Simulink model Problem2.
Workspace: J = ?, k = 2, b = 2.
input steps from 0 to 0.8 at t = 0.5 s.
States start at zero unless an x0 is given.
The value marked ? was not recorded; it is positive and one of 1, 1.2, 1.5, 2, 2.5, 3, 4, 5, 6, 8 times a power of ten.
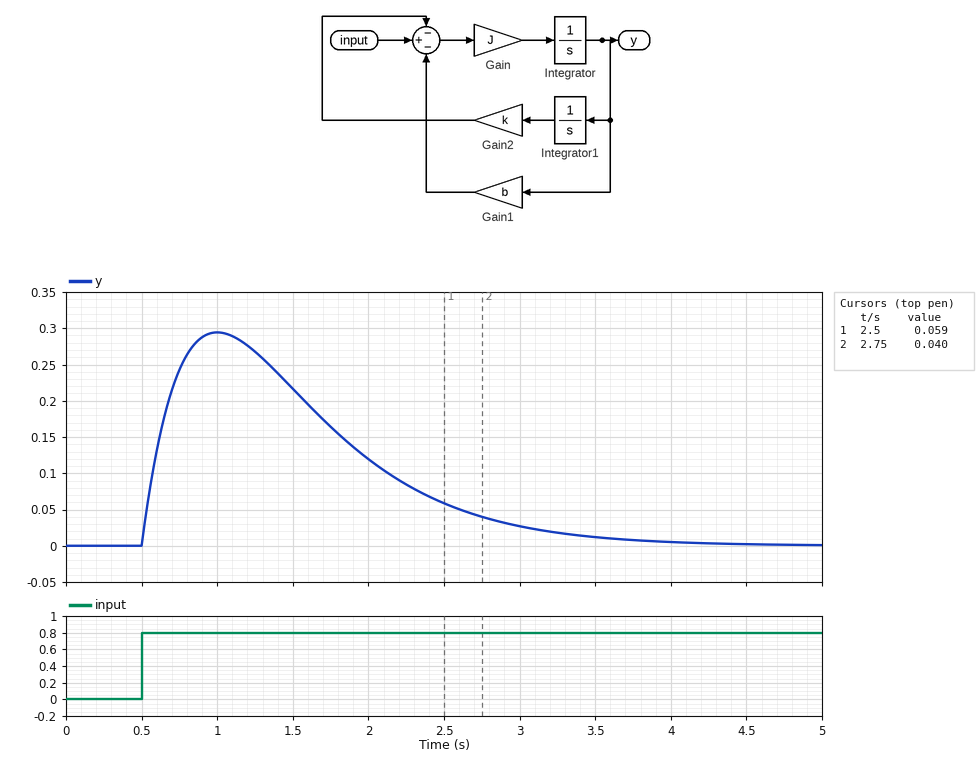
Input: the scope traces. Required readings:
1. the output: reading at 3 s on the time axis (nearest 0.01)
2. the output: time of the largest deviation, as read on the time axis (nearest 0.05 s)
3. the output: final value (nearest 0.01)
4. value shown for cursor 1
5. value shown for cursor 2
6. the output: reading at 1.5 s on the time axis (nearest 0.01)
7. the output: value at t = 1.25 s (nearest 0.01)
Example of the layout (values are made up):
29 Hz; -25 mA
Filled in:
0.03; 1.00 s; 0.00; 0.059; 0.040; 0.22; 0.27
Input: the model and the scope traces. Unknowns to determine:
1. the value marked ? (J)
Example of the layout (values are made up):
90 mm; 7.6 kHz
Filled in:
2
